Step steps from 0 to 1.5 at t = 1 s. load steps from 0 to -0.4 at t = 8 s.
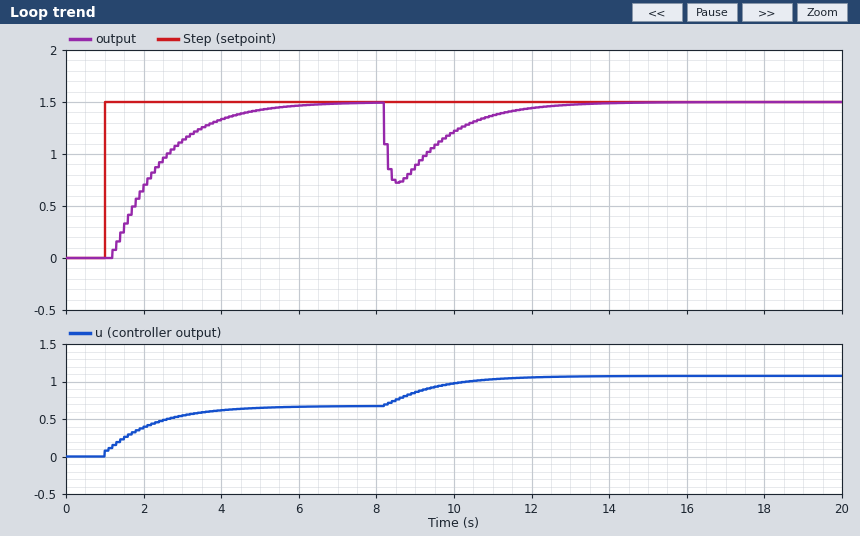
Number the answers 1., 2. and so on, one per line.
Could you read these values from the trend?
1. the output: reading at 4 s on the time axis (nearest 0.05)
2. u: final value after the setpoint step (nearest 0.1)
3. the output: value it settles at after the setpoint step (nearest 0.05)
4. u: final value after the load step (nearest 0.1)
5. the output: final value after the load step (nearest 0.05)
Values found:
1. 1.35
2. 0.7
3. 1.50
4. 1.1
5. 1.50
